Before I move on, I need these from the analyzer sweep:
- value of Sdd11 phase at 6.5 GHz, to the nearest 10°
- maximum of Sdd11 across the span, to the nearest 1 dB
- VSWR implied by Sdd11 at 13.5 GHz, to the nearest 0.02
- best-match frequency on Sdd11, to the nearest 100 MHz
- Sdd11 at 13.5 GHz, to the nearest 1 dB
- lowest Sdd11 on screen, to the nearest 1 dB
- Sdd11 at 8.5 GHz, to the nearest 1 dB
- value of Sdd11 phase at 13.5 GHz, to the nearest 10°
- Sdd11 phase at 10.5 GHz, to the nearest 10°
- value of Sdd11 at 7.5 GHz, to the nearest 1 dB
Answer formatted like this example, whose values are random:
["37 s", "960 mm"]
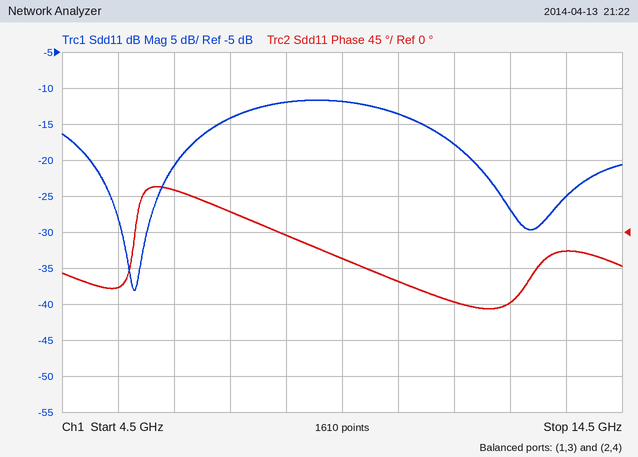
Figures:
["50°", "-12 dB", "1.12", "5.8 GHz", "-25 dB", "-38 dB", "-12 dB", "-20°", "-60°", "-14 dB"]
